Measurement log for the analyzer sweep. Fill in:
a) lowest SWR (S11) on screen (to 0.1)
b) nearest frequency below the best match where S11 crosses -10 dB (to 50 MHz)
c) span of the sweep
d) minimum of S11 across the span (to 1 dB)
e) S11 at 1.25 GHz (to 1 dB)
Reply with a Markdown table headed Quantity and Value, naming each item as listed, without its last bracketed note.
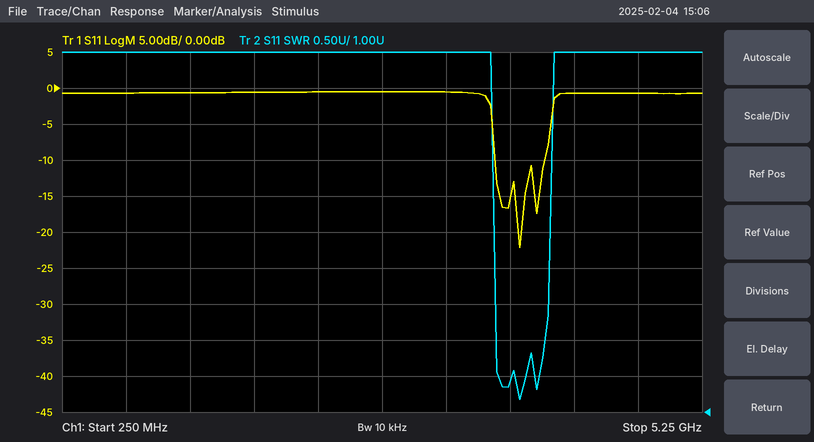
| Quantity | Value |
|---|---|
| lowest SWR (S11) on screen | 1.2 |
| nearest frequency below the best match where S11 crosses -10 dB | 3.65 GHz |
| span of the sweep | 5 GHz |
| minimum of S11 across the span | -22 dB |
| S11 at 1.25 GHz | -1 dB |
